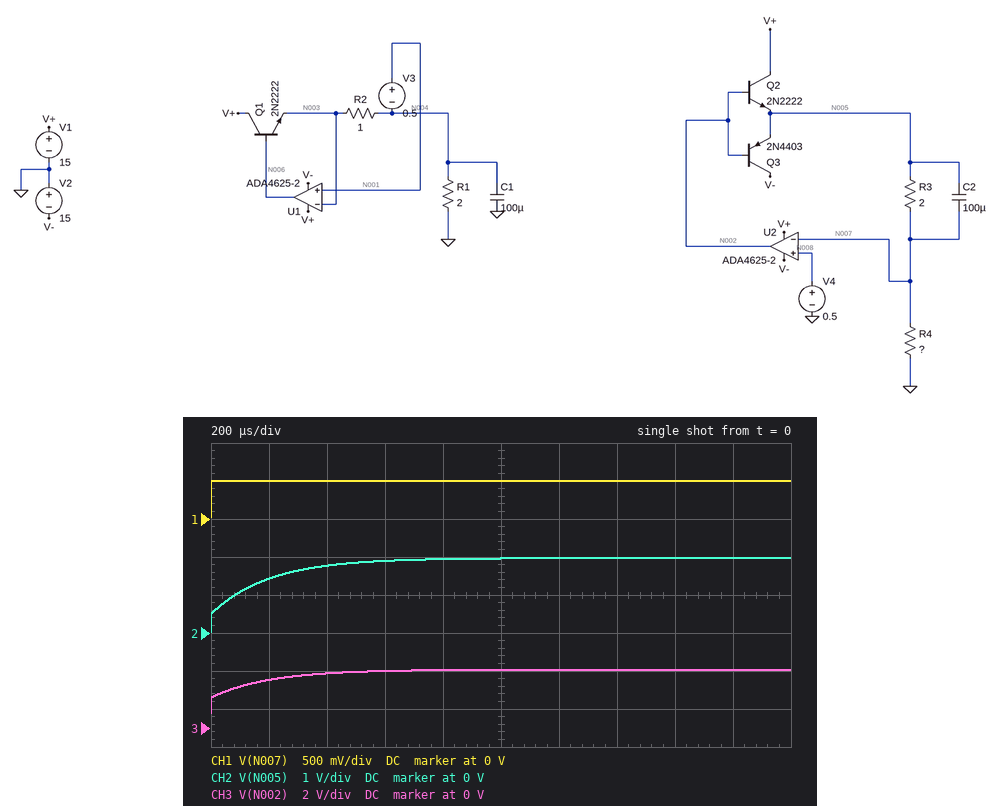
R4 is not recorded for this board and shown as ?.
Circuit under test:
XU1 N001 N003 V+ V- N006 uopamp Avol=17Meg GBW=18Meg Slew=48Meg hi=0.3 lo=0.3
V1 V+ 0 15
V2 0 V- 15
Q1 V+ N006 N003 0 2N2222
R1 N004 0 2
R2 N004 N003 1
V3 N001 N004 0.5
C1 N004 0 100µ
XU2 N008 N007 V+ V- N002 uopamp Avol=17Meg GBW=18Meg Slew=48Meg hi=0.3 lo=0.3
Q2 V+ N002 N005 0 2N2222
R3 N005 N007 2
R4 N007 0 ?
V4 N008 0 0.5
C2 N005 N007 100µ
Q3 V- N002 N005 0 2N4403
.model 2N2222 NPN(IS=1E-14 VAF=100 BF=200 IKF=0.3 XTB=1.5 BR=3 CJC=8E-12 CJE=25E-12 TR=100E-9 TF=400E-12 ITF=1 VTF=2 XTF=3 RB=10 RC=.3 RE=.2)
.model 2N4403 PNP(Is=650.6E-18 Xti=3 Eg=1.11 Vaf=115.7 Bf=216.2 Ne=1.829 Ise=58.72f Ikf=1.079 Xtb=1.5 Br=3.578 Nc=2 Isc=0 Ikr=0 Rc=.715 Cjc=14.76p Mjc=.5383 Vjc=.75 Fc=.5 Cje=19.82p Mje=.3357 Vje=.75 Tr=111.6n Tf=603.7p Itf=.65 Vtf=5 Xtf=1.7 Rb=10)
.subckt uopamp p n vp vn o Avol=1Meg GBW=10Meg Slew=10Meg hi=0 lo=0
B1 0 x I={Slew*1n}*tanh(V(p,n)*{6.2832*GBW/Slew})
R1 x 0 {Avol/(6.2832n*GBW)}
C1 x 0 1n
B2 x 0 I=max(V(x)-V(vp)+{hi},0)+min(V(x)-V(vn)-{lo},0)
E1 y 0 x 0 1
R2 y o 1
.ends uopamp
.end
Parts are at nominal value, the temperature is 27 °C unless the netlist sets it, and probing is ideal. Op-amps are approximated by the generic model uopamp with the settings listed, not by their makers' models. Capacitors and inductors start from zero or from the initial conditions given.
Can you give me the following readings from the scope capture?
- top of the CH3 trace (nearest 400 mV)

3.2 V
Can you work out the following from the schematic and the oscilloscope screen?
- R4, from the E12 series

0.68 Ω
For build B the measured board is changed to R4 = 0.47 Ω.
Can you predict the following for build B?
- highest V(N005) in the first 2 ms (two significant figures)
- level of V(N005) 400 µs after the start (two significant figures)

2.6 V
2.3 V
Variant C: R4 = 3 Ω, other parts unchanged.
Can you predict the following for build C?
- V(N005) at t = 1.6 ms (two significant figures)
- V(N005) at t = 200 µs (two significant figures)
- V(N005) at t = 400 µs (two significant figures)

830 mV
710 mV
790 mV
